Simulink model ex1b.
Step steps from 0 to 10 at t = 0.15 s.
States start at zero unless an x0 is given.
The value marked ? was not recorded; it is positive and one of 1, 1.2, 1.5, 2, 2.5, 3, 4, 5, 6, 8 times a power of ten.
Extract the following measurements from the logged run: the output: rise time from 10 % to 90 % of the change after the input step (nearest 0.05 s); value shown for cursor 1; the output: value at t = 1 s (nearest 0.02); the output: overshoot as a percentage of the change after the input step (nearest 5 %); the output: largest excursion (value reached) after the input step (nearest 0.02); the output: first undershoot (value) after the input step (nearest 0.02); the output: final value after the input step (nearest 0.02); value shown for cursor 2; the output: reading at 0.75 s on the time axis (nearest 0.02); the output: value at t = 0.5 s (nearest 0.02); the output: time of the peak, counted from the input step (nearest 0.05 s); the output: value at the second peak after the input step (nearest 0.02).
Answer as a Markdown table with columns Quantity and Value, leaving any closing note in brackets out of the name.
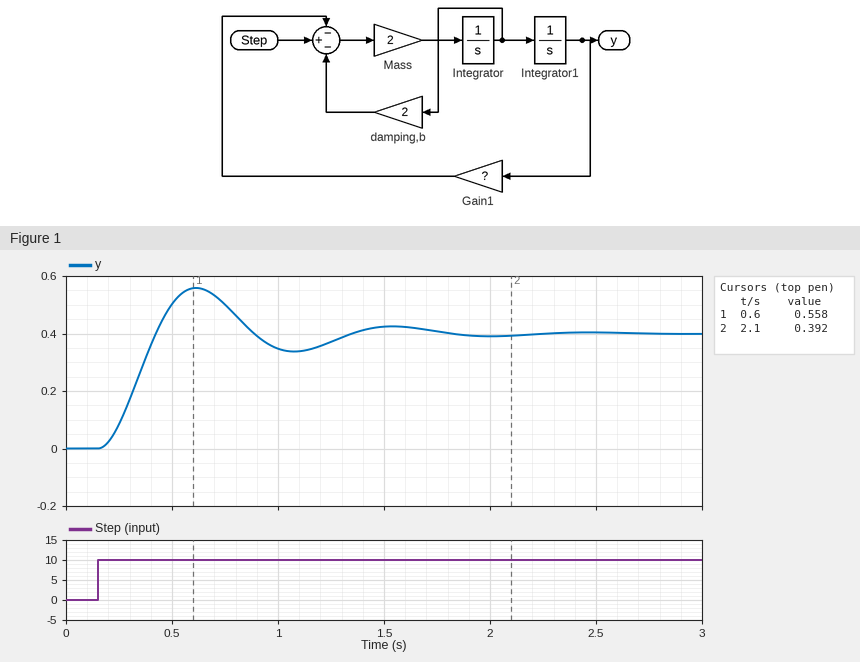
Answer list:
| Quantity | Value |
|---|---|
| the output: rise time from 10 % to 90 % of the change after the input step | 0.20 s |
| value shown for cursor 1 | 0.558 |
| the output: value at t = 1 s | 0.34 |
| the output: overshoot as a percentage of the change after the input step | 40 % |
| the output: largest excursion (value reached) after the input step | 0.56 |
| the output: first undershoot (value) after the input step | 0.34 |
| the output: final value after the input step | 0.40 |
| value shown for cursor 2 | 0.392 |
| the output: reading at 0.75 s on the time axis | 0.50 |
| the output: value at t = 0.5 s | 0.50 |
| the output: time of the peak, counted from the input step | 0.45 s |
| the output: value at the second peak after the input step | 0.42 |
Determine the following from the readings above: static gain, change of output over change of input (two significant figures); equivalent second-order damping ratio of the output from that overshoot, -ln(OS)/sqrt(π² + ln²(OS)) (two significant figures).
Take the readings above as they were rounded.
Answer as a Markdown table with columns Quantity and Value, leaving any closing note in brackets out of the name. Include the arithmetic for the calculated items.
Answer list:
| Quantity | Value |
|---|---|
| static gain, change of output over change of input | (0.4 - 0) / (10 - 0) = 0.040 |
| equivalent second-order damping ratio of the output from that overshoot, -ln(OS)/sqrt(π² + ln²(OS)) | ln(0.4) = -0.916; 0.916 / sqrt(9.870 + 0.840) = 0.28 |
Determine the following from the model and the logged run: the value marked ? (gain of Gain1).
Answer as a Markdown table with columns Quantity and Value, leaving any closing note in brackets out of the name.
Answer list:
| Quantity | Value |
|---|---|
| the value marked ? | 25 |
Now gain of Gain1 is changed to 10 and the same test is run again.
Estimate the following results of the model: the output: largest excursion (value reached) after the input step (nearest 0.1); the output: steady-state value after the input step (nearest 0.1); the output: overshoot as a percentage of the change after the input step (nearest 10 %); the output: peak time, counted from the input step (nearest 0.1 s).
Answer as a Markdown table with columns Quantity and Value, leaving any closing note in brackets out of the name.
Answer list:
| Quantity | Value |
|---|---|
| the output: largest excursion (value reached) after the input step | 1.2 |
| the output: steady-state value after the input step | 1.0 |
| the output: overshoot as a percentage of the change after the input step | 20 % |
| the output: peak time, counted from the input step | 0.8 s |
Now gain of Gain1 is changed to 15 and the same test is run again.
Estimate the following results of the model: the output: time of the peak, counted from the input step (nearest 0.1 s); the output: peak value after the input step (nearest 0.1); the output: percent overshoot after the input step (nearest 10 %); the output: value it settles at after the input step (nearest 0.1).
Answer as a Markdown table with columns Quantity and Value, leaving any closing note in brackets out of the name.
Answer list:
| Quantity | Value |
|---|---|
| the output: time of the peak, counted from the input step | 0.6 s |
| the output: peak value after the input step | 0.9 |
| the output: percent overshoot after the input step | 30 % |
| the output: value it settles at after the input step | 0.7 |
